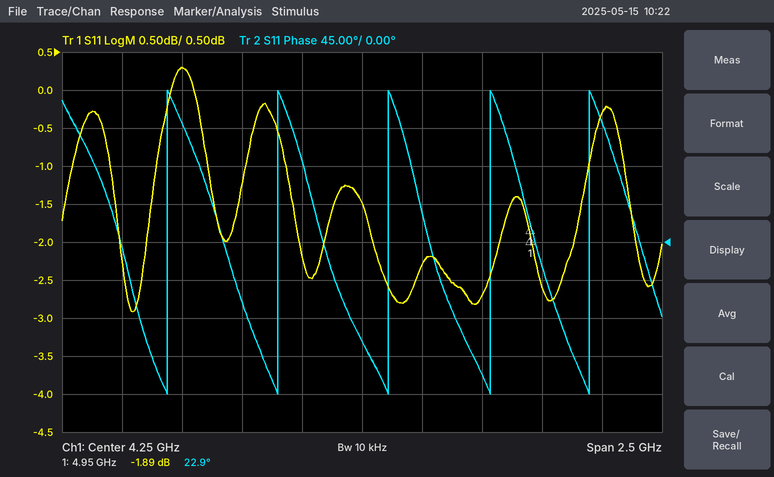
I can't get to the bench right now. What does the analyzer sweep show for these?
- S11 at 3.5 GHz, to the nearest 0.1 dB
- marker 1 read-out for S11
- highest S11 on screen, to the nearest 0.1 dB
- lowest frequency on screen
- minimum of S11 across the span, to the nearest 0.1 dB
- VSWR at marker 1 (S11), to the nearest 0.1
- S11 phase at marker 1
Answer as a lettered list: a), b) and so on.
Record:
a) 0.3 dB
b) -1.89 dB
c) 0.3 dB
d) 3 GHz
e) -2.9 dB
f) 9.2
g) 22.9°
